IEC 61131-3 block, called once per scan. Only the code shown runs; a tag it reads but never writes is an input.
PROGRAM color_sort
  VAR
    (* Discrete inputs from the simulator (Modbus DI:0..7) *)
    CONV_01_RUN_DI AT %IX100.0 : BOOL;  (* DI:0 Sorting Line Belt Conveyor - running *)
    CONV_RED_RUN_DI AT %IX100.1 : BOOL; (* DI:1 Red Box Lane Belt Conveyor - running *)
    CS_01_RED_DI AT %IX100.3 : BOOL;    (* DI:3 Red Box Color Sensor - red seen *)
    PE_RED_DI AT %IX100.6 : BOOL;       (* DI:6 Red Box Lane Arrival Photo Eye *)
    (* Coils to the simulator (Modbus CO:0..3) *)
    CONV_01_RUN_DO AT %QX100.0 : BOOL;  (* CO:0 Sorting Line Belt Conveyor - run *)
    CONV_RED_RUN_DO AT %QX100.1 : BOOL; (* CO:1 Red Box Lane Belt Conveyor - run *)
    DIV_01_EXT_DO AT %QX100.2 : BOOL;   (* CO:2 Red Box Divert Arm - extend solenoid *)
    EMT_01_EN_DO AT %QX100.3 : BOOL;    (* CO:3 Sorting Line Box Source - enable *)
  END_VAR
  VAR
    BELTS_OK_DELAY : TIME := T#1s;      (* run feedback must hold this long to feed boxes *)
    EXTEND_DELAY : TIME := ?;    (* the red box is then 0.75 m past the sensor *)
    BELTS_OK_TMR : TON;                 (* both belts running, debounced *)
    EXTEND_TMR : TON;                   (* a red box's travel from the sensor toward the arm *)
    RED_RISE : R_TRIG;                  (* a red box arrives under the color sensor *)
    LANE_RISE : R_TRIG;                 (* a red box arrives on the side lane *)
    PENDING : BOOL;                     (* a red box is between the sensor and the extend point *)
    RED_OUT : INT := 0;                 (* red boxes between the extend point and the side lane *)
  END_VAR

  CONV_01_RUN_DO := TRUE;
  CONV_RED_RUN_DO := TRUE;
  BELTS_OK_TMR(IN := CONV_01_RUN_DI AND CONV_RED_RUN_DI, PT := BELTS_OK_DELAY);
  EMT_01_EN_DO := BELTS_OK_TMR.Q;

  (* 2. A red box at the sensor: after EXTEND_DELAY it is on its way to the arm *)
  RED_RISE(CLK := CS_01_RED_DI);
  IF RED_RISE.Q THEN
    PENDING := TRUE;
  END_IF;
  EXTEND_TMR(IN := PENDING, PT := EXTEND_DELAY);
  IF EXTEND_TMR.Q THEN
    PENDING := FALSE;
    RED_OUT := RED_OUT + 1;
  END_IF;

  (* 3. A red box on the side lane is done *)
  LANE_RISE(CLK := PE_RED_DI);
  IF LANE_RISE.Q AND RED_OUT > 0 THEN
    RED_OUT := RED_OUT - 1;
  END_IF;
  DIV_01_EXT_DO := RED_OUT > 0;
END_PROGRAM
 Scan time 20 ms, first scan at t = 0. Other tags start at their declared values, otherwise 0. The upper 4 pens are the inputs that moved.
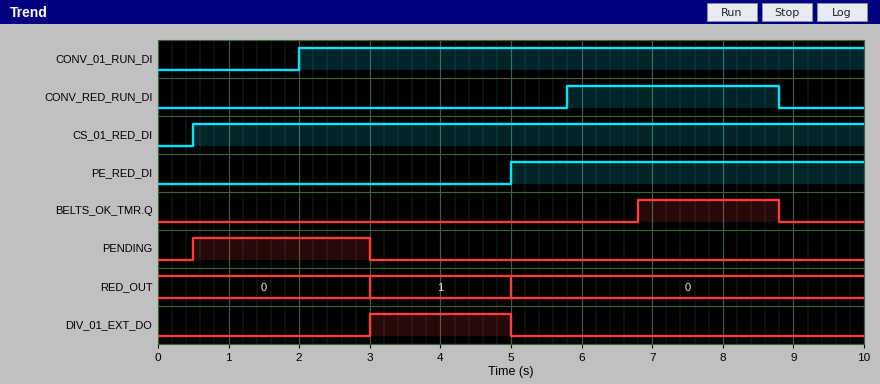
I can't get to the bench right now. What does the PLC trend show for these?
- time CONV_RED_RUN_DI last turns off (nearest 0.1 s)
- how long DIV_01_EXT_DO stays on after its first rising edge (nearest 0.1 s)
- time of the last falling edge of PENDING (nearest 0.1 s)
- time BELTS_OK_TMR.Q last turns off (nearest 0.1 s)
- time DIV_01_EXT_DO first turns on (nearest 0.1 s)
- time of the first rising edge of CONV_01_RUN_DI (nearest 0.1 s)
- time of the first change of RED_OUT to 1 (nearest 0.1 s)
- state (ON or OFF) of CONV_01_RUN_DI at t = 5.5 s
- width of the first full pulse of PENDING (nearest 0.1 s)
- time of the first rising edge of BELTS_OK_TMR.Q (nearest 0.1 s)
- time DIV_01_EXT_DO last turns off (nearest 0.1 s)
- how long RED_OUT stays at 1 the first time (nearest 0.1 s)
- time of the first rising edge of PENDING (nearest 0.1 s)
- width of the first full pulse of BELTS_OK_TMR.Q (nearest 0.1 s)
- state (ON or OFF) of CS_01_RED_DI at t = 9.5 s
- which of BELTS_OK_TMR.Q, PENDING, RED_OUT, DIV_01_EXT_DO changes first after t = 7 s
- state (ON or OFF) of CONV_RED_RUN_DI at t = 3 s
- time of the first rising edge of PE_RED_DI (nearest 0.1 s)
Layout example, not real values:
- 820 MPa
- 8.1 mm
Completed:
- 8.8 s
- 2.0 s
- 3.0 s
- 8.8 s
- 3.0 s
- 2.0 s
- 3.0 s
- ON
- 2.5 s
- 6.8 s
- 5.0 s
- 2.0 s
- 0.5 s
- 2.0 s
- ON
- BELTS_OK_TMR.Q
- OFF
- 5.0 s
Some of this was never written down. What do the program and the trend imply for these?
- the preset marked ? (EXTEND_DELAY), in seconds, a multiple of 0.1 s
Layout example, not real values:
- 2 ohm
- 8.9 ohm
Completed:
- 2.5 s
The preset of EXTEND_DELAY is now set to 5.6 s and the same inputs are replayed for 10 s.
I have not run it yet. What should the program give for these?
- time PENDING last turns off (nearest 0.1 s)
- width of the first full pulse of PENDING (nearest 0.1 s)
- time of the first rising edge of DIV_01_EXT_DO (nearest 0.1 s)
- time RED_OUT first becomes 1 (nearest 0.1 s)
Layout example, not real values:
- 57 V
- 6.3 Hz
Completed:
- 6.1 s
- 5.6 s
- 6.1 s
- 6.1 s
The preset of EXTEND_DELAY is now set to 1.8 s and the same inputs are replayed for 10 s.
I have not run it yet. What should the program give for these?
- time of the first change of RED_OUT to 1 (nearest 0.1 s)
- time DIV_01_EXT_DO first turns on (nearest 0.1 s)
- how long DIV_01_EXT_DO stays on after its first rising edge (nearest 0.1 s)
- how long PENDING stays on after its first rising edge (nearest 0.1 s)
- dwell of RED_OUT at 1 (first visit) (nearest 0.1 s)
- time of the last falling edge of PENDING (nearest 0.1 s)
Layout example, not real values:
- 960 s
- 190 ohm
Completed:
- 2.3 s
- 2.3 s
- 2.7 s
- 1.8 s
- 2.7 s
- 2.3 s
